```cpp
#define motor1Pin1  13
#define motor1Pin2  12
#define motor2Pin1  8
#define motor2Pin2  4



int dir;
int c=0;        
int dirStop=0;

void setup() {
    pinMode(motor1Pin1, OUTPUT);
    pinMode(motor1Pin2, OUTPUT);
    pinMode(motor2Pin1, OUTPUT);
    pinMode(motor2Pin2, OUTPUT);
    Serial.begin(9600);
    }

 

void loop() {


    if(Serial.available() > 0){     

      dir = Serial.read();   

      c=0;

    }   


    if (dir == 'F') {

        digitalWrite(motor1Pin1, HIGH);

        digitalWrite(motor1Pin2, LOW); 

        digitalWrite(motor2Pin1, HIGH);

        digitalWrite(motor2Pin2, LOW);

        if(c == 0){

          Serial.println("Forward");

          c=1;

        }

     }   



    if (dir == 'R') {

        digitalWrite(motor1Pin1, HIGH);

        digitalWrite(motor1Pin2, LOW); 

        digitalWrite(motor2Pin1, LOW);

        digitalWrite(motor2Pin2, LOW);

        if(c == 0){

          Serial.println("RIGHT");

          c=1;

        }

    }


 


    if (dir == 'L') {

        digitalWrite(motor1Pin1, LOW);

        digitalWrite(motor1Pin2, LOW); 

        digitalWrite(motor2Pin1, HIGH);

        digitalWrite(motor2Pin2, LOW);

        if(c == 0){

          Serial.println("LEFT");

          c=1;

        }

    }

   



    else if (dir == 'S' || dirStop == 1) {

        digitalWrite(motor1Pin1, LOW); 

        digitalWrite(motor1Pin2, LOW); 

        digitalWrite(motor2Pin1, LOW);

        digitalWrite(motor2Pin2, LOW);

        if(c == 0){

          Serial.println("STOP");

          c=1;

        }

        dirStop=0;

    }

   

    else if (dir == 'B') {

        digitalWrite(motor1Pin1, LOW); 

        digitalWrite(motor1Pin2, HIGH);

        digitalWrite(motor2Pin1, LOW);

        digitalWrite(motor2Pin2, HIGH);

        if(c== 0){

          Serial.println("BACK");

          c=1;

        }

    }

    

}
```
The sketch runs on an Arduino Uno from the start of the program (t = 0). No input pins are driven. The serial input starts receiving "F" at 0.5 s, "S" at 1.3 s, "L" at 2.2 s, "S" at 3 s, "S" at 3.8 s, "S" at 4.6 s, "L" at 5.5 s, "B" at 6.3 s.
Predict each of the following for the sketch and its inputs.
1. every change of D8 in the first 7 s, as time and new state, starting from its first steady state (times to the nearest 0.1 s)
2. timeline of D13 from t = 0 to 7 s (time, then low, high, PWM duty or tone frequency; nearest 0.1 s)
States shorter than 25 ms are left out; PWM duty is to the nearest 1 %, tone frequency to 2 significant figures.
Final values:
0 s low; 0.5 s high; 1.3 s low; 2.2 s high; 3 s low; 5.5 s high; 6.3 s low
0 s low; 0.5 s high; 1.3 s low
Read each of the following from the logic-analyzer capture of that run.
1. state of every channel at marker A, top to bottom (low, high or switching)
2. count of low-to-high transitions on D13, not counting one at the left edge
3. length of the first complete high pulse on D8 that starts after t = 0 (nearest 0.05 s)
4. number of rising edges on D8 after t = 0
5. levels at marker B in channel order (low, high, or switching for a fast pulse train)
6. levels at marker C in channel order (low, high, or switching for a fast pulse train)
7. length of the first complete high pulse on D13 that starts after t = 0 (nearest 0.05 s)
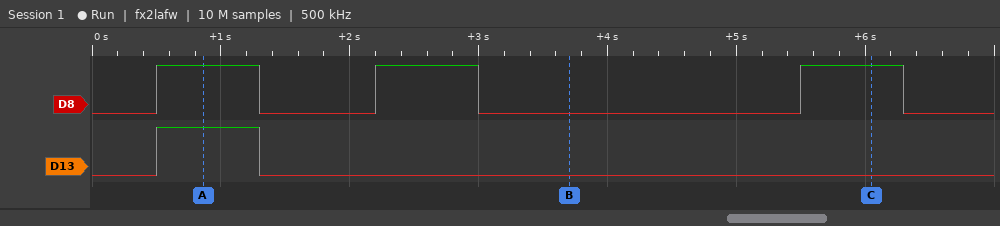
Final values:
D8 high, D13 high
1
0.80 s
3
D8 low, D13 low
D8 high, D13 low
0.80 s
